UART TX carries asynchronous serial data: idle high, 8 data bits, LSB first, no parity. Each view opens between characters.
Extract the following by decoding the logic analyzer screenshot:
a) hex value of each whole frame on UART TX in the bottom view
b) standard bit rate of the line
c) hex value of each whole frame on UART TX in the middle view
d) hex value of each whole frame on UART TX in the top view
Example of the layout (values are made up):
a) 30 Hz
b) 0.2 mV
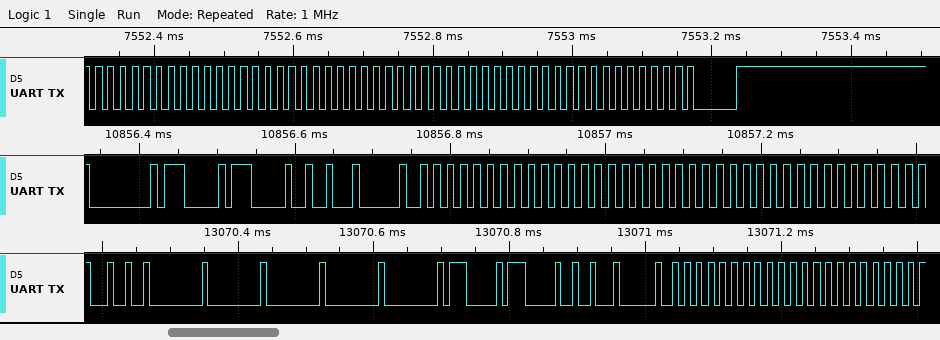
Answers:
a) 24, 00, 00, 00, 00, 00, 07, 07, 12, 20, 55, 55, 55, 55
b) 115200 baud
c) 00, 07, 07, 12, 20, 55, 55, 55, 55, 55, 55, 55
d) 55, 55, 55, 55, 55, 55, 55, 55, 55, 55, C0
